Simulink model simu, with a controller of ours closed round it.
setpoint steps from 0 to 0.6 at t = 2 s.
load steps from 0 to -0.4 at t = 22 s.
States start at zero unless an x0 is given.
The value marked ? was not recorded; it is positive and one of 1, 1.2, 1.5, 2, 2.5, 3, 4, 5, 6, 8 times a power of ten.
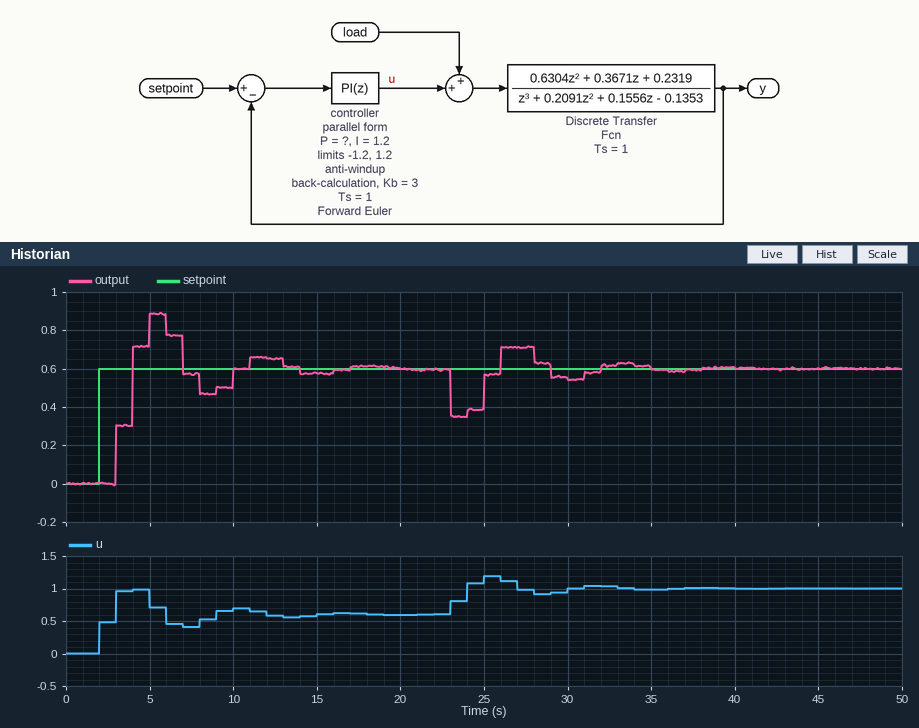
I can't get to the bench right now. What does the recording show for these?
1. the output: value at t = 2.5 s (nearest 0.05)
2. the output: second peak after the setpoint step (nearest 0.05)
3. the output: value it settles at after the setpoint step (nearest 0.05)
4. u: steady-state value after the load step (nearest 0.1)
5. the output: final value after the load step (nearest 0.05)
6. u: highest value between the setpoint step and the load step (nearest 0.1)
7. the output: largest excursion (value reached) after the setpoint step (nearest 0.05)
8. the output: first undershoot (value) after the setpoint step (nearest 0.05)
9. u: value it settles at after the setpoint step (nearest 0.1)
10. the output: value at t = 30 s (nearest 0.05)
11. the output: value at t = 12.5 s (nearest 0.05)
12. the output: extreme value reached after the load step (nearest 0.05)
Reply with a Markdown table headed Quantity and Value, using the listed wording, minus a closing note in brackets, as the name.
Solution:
| Quantity | Value |
|---|---|
| the output: value at t = 2.5 s | 0.00 |
| the output: second peak after the setpoint step | 0.65 |
| the output: value it settles at after the setpoint step | 0.60 |
| u: steady-state value after the load step | 1.0 |
| the output: final value after the load step | 0.60 |
| u: highest value between the setpoint step and the load step | 1.0 |
| the output: largest excursion (value reached) after the setpoint step | 0.90 |
| the output: first undershoot (value) after the setpoint step | 0.45 |
| u: value it settles at after the setpoint step | 0.6 |
| the output: value at t = 30 s | 0.55 |
| the output: value at t = 12.5 s | 0.65 |
| the output: extreme value reached after the load step | 0.35 |
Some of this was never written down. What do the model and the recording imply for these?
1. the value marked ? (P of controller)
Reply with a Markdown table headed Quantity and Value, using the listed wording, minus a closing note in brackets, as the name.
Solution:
| Quantity | Value |
|---|---|
| the value marked ? | 0.8 |
